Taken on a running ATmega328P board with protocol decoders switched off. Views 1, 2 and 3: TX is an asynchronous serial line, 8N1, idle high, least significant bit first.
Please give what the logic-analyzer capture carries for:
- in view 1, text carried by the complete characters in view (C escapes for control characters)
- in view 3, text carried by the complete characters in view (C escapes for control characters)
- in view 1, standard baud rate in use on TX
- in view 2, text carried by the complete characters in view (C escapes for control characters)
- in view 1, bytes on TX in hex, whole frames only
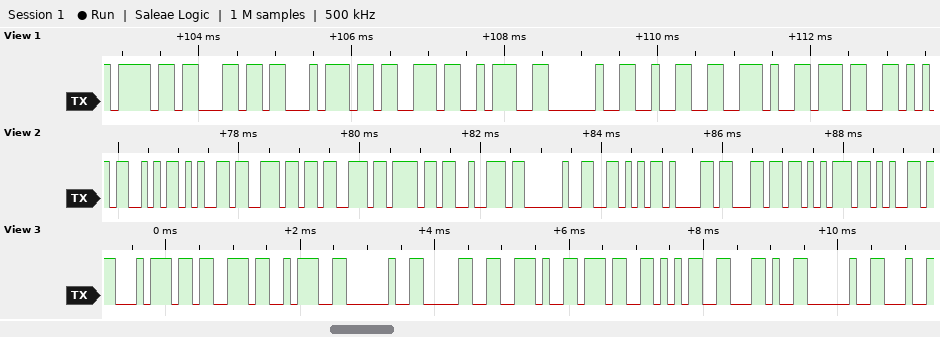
"olts: 2.7"
"ts: 0.75, "
9600 baud
"Sensor Value"
0x6F 0x6C 0x74 0x73 0x3A 0x20 0x32 0x2E 0x37
